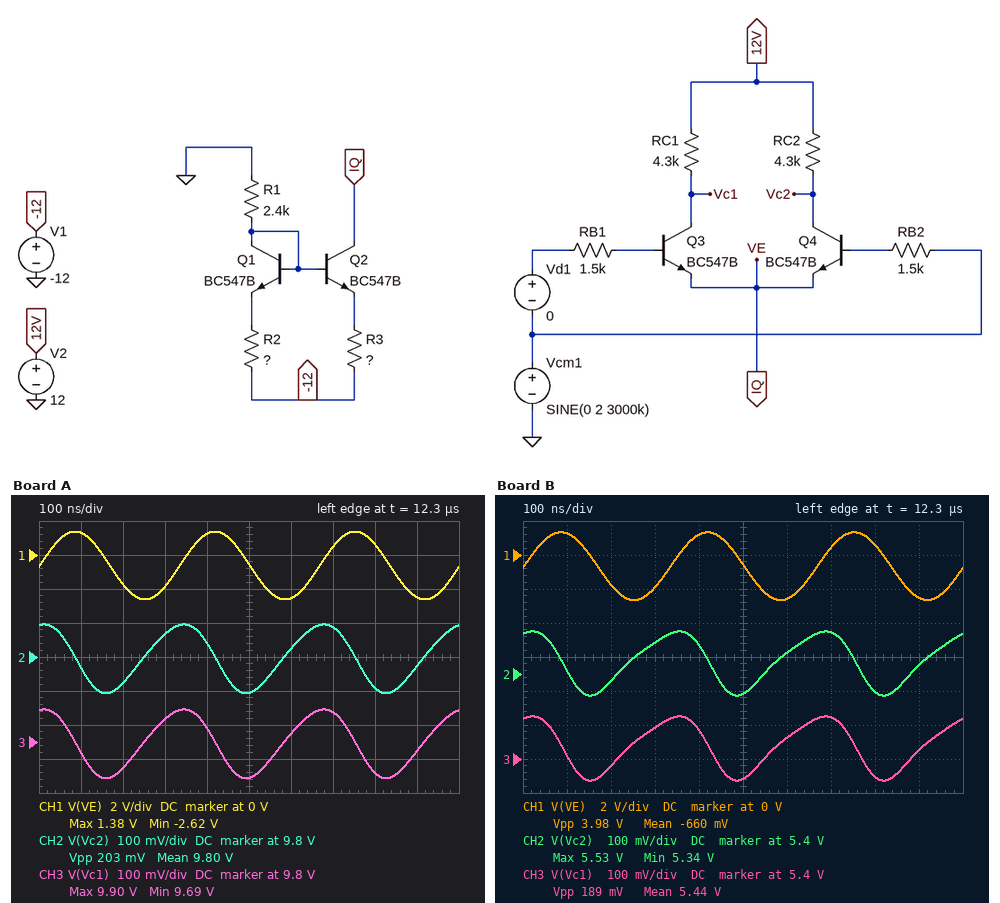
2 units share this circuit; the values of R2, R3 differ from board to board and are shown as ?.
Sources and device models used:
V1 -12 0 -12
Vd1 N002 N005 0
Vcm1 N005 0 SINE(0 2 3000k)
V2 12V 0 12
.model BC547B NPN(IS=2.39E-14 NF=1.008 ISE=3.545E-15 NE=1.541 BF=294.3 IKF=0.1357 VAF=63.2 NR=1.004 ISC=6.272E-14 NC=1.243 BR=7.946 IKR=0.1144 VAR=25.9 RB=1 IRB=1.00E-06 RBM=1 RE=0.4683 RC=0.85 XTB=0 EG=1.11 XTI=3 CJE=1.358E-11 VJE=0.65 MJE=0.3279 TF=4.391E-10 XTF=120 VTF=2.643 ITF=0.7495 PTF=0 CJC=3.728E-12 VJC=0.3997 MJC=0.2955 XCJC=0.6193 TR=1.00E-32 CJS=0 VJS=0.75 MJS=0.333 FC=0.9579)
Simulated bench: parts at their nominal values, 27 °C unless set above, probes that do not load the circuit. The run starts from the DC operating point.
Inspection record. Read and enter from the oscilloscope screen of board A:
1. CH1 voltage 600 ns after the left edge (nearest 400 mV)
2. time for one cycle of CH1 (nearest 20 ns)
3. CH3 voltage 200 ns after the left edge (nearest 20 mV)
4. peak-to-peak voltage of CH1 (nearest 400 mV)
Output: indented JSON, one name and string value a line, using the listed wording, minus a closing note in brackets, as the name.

{
  "CH1 voltage 600 ns after the left edge": "-2.4 V",
  "time for one cycle of CH1": "340 ns",
  "CH3 voltage 200 ns after the left edge": "9.72 V",
  "peak-to-peak voltage of CH1": "4.0 V"
}
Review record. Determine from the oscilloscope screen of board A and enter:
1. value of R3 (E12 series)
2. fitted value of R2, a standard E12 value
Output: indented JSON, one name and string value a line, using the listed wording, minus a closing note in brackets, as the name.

{
  "value of R3": "220 Ω",
  "fitted value of R2, a standard E12 value": "39 Ω"
}
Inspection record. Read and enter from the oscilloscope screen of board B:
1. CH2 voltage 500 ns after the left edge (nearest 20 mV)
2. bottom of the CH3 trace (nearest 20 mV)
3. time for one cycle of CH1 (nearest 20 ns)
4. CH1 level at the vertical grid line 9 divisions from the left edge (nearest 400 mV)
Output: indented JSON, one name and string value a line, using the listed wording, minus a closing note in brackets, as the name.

{
  "CH2 voltage 500 ns after the left edge": "5.34 V",
  "bottom of the CH3 trace": "5.34 V",
  "time for one cycle of CH1": "340 ns",
  "CH1 level at the vertical grid line 9 divisions from the left edge": "-2.4 V"
}
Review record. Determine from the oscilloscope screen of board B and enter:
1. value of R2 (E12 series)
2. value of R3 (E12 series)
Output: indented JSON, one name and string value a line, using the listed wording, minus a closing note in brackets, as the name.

{
  "value of R2": "120 Ω",
  "value of R3": "180 Ω"
}
